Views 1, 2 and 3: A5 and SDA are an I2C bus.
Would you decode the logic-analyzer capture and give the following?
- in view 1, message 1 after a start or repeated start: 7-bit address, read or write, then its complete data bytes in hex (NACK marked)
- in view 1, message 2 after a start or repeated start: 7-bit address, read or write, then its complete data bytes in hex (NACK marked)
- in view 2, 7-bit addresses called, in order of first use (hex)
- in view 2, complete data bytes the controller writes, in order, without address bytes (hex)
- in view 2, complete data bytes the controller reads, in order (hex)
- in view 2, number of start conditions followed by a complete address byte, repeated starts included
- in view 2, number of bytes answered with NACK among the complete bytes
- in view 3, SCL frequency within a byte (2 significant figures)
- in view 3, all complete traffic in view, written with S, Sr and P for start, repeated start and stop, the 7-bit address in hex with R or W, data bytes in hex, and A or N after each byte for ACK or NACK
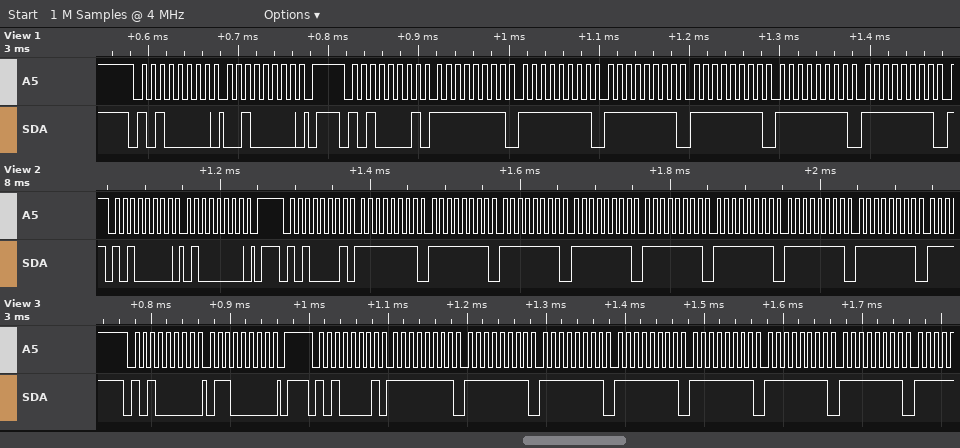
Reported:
0x50 write: 20
0x50 read: FF FF FF FF FF FF
0x50
40
FF FF FF FF FF FF FF FF
2
0
100 kHz
S 50W A 60 A P S 50R A FF A FF A FF A FF A FF A FF A FF A
